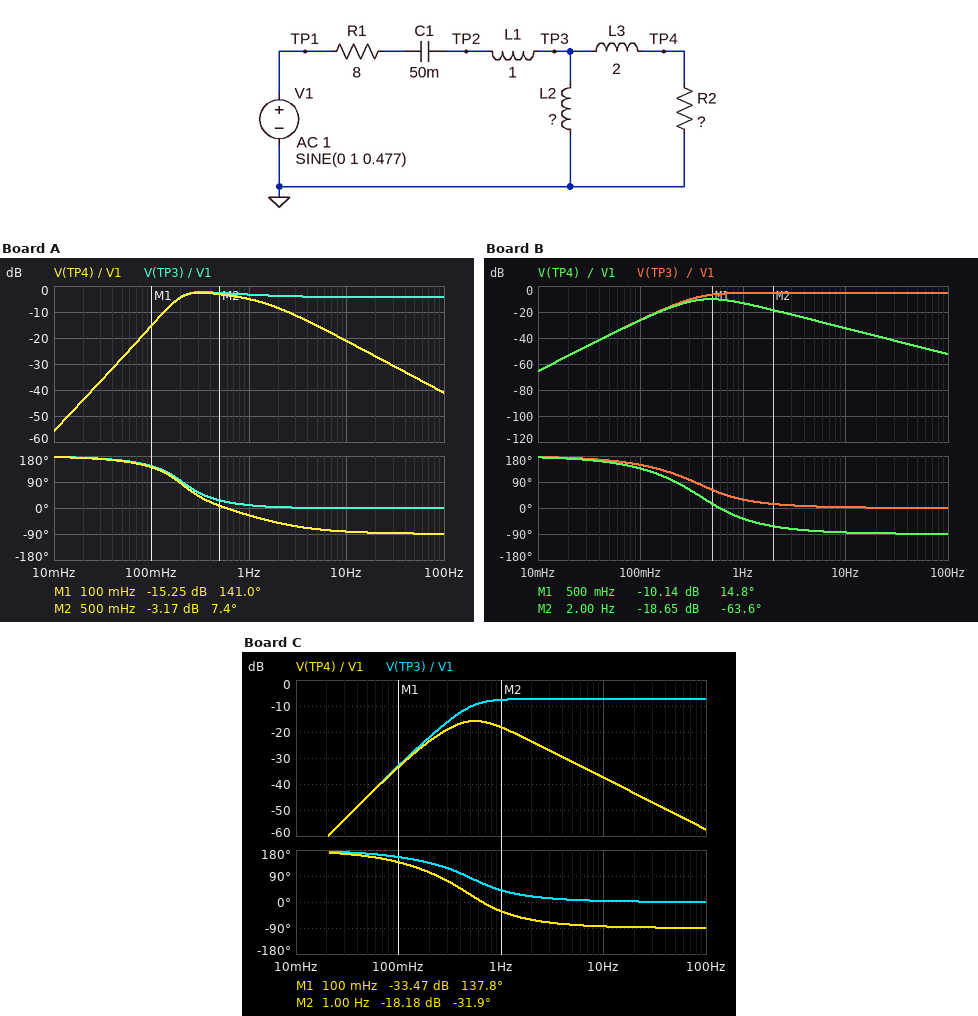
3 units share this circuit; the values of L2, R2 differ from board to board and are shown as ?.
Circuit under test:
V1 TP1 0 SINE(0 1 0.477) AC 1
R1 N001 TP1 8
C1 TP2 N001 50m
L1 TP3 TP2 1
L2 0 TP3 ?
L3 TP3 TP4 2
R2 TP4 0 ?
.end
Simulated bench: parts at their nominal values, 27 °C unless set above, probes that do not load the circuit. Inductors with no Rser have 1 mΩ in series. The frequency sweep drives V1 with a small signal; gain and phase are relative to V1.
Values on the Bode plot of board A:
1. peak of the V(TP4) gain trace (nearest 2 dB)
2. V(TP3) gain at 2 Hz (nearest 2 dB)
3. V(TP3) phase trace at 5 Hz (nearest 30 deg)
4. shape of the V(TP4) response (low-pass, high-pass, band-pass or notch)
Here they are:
-2 dB
-4 dB
0 deg
band-pass
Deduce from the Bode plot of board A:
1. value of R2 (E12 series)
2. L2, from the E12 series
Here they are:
18 Ω
8.2 H
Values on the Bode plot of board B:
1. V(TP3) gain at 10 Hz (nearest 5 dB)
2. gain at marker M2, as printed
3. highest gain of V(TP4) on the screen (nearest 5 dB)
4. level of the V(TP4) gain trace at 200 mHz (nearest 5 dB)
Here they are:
-5 dB
-18.65 dB
-10 dB
-15 dB
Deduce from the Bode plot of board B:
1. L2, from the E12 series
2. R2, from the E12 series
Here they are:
2.7 H
5.6 Ω
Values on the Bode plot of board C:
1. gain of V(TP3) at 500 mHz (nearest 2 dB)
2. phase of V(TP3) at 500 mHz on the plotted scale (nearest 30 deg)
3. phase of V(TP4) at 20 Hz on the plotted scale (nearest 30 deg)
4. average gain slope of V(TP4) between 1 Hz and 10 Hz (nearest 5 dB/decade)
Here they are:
-10 dB
90 deg
-90 deg
-20 dB/decade
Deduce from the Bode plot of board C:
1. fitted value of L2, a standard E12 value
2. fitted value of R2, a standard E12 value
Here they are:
1.2 H
3.9 Ω
